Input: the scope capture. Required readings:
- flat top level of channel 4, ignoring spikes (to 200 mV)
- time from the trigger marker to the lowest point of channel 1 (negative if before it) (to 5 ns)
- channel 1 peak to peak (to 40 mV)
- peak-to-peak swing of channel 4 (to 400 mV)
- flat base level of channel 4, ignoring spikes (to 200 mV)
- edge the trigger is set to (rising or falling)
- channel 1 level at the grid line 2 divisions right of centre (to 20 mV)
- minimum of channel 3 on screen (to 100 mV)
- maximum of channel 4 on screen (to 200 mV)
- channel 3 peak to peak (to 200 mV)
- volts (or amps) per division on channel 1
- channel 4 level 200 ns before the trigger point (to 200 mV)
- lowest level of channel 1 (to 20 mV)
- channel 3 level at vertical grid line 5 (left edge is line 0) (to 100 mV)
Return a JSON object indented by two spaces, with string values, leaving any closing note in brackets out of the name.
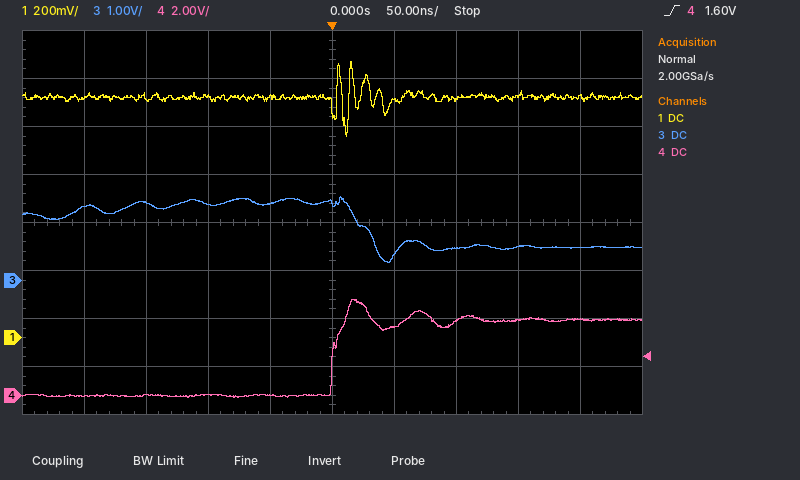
{
  "flat top level of channel 4, ignoring spikes": "3.2 V",
  "time from the trigger marker to the lowest point of channel 1 (negative if before it)": "+10 ns",
  "channel 1 peak to peak": "320 mV",
  "peak-to-peak swing of channel 4": "4.0 V",
  "flat base level of channel 4, ignoring spikes": "0.0 V",
  "edge the trigger is set to": "rising",
  "channel 1 level at the grid line 2 divisions right of centre": "1.00 V",
  "minimum of channel 3 on screen": "400 mV",
  "maximum of channel 4 on screen": "4.0 V",
  "channel 3 peak to peak": "1.4 V",
  "volts (or amps) per division on channel 1": "200 mV",
  "channel 4 level 200 ns before the trigger point": "0.0 V",
  "lowest level of channel 1": "840 mV",
  "channel 3 level at vertical grid line 5 (left edge is line 0)": "1.6 V"
}
